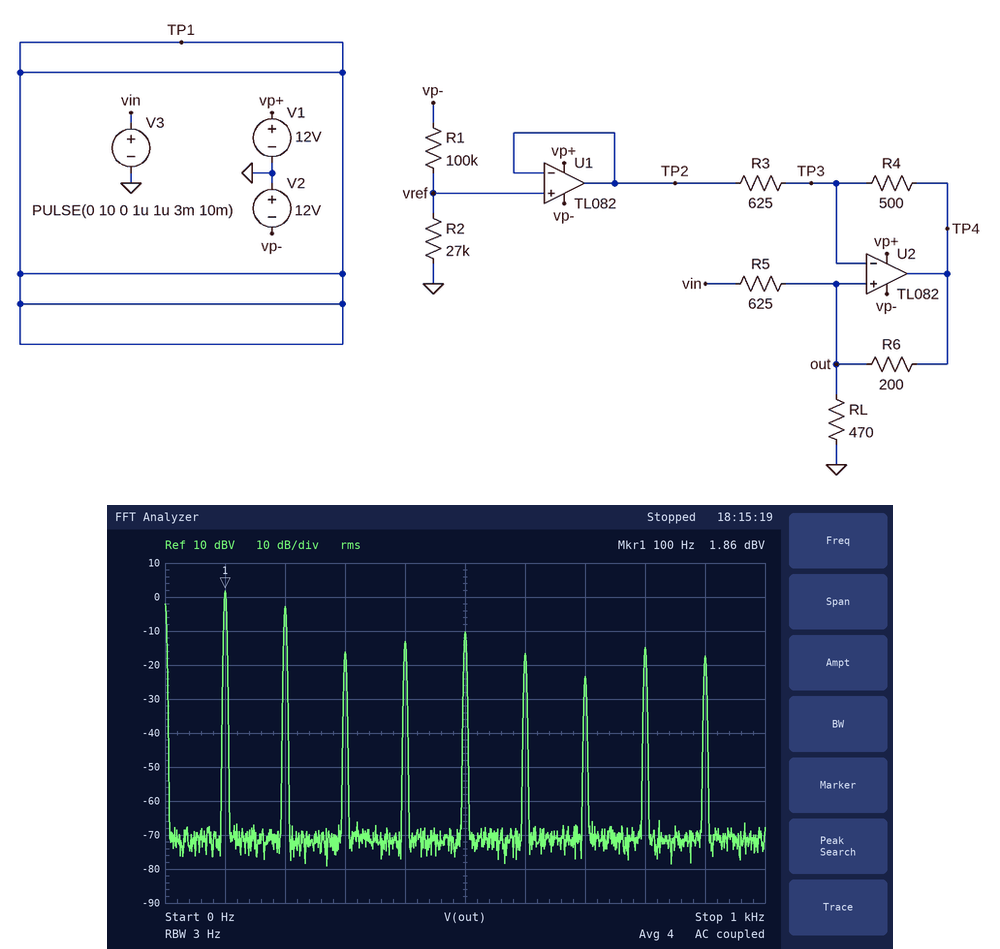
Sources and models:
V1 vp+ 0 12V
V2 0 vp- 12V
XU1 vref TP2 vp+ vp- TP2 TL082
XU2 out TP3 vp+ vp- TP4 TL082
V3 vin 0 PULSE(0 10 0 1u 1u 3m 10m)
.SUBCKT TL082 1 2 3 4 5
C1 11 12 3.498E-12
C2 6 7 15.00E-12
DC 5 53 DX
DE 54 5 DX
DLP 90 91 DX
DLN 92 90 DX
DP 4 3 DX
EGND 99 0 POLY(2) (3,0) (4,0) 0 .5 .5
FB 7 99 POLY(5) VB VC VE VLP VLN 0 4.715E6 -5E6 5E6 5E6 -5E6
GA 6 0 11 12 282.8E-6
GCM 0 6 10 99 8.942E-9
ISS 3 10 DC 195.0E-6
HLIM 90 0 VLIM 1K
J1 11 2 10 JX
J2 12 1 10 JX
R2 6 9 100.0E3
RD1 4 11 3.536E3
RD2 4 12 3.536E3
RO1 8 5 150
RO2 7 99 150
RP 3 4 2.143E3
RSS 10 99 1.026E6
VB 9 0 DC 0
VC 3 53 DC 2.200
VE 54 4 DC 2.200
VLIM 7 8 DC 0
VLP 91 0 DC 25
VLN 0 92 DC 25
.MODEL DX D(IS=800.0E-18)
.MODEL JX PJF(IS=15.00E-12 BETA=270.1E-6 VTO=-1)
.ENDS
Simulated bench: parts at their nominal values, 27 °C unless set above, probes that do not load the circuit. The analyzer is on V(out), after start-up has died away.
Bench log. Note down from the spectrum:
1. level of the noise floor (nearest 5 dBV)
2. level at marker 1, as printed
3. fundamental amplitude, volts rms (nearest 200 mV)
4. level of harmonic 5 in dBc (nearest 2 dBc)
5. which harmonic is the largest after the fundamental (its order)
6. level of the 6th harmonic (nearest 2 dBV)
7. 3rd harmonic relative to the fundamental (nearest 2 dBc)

-70 dBV
1.86 dBV
1.2 V
-12 dBc
2
-16 dBV
-18 dBc
